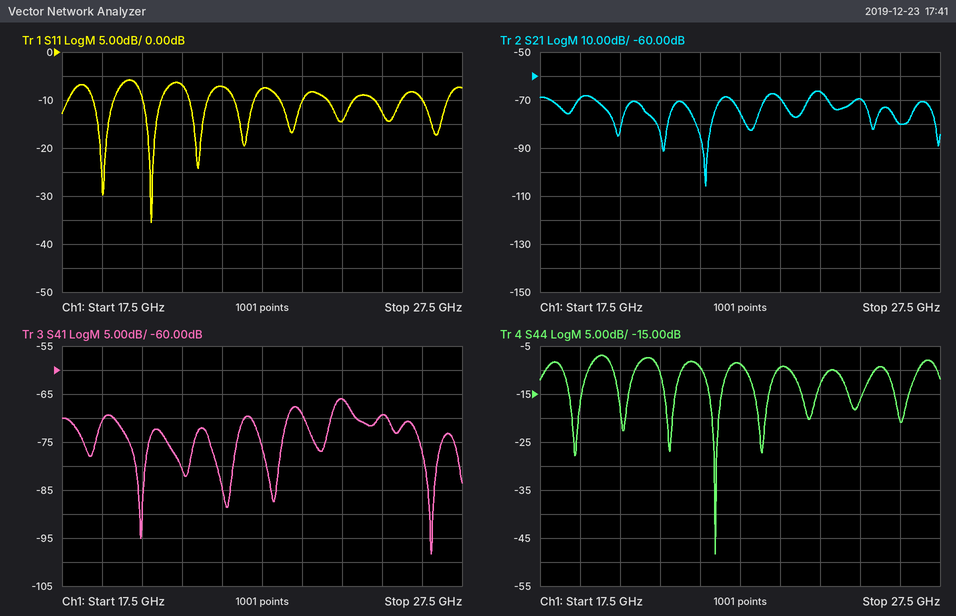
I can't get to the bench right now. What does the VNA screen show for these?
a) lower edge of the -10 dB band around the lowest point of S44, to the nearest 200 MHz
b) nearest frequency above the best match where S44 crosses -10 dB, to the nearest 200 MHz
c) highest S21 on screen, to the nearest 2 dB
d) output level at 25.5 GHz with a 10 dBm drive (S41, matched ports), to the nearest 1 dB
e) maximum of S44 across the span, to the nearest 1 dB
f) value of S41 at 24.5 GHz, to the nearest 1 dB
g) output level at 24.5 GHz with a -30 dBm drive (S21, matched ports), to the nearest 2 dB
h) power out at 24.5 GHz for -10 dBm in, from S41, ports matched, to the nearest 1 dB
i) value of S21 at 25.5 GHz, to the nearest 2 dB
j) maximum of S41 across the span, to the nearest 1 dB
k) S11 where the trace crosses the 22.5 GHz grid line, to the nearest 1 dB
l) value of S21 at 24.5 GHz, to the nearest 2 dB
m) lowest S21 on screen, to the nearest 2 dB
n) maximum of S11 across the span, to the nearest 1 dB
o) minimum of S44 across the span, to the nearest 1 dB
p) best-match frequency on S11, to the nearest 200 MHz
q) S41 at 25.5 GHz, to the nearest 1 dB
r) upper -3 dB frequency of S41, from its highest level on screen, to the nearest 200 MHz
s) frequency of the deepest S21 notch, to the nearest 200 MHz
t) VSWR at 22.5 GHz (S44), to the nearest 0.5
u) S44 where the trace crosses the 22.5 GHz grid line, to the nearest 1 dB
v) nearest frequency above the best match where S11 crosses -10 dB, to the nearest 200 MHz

21.6 GHz
22.2 GHz
-66 dB
-59 dBm
-7 dB
-66 dB
-96 dBm
-76 dBm
-70 dB
-66 dB
-8 dB
-66 dB
-106 dB
-6 dB
-48 dB
19.8 GHz
-69 dB
24.8 GHz
21.6 GHz
2.0
-9 dB
20.0 GHz
